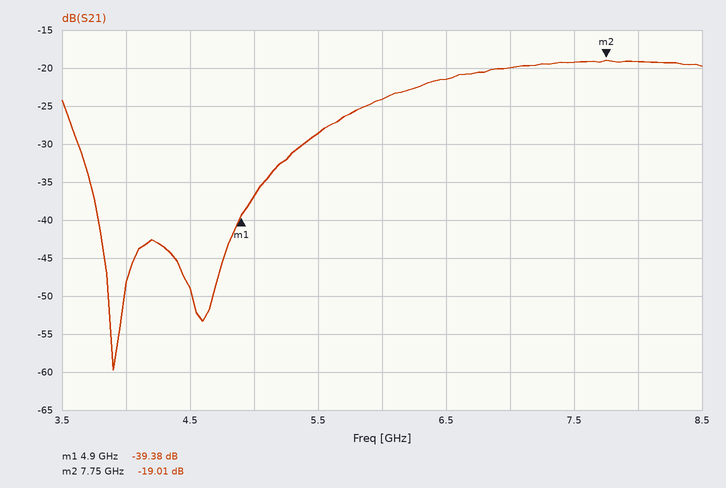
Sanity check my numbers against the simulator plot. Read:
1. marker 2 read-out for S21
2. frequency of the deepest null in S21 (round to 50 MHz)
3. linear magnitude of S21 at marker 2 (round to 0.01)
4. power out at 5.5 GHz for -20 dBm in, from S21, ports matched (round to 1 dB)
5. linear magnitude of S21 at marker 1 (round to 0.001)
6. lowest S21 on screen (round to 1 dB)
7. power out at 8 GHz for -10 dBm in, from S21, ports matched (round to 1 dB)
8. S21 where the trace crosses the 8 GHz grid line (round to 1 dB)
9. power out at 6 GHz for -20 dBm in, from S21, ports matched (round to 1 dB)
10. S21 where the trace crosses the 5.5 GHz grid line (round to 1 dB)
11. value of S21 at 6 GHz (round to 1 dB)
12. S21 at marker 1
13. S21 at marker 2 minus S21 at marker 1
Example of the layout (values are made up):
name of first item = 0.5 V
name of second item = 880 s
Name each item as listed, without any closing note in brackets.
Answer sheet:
marker 2 read-out for S21 = -19.01 dB
frequency of the deepest null in S21 = 3.90 GHz
linear magnitude of S21 at marker 2 = 0.11
power out at 5.5 GHz for -20 dBm in, from S21, ports matched = -49 dBm
linear magnitude of S21 at marker 1 = 0.011
lowest S21 on screen = -60 dB
power out at 8 GHz for -10 dBm in, from S21, ports matched = -29 dBm
S21 where the trace crosses the 8 GHz grid line = -19 dB
power out at 6 GHz for -20 dBm in, from S21, ports matched = -44 dBm
S21 where the trace crosses the 5.5 GHz grid line = -29 dB
value of S21 at 6 GHz = -24 dB
S21 at marker 1 = -39.38 dB
S21 at marker 2 minus S21 at marker 1 = 20.37 dB
